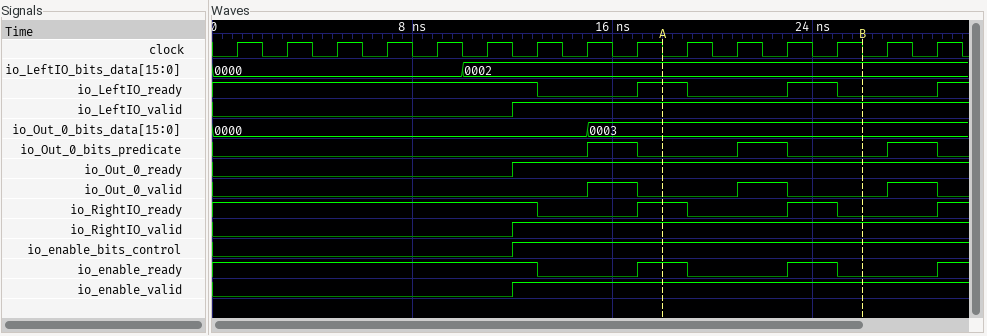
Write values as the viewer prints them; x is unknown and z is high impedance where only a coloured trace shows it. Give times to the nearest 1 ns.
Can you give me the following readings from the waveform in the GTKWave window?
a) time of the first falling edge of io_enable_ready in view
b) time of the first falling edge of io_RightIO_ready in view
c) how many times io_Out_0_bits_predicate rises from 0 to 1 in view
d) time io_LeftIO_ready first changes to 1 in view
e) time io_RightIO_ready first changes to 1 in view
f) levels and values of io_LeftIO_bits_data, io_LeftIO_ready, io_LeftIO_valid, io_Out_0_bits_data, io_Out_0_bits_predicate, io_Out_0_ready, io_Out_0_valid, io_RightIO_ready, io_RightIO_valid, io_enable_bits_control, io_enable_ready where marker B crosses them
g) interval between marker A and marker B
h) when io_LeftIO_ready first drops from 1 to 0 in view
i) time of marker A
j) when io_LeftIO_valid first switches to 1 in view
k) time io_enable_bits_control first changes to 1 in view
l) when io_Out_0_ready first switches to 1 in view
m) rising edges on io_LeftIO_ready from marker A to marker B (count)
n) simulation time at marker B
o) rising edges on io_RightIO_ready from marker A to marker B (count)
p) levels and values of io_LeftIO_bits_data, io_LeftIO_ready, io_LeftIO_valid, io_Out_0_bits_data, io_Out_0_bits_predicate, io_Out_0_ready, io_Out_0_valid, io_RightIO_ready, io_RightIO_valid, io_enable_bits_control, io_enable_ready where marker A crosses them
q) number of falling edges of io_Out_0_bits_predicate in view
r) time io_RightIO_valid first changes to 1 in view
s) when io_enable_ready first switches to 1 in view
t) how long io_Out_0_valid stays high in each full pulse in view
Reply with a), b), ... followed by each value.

a) 13 ns
b) 13 ns
c) 3
d) 17 ns
e) 17 ns
f) io_LeftIO_bits_data=0002, io_LeftIO_ready=0, io_LeftIO_valid=1, io_Out_0_bits_data=0003, io_Out_0_bits_predicate=0, io_Out_0_ready=1, io_Out_0_valid=0, io_RightIO_ready=0, io_RightIO_valid=1, io_enable_bits_control=1, io_enable_ready=0
g) 8 ns
h) 13 ns
i) 18 ns
j) 12 ns
k) 12 ns
l) 12 ns
m) 1
n) 26 ns
o) 1
p) io_LeftIO_bits_data=0002, io_LeftIO_ready=1, io_LeftIO_valid=1, io_Out_0_bits_data=0003, io_Out_0_bits_predicate=0, io_Out_0_ready=1, io_Out_0_valid=0, io_RightIO_ready=1, io_RightIO_valid=1, io_enable_bits_control=1, io_enable_ready=1
q) 3
r) 12 ns
s) 17 ns
t) 2 ns, 2 ns, 2 ns
